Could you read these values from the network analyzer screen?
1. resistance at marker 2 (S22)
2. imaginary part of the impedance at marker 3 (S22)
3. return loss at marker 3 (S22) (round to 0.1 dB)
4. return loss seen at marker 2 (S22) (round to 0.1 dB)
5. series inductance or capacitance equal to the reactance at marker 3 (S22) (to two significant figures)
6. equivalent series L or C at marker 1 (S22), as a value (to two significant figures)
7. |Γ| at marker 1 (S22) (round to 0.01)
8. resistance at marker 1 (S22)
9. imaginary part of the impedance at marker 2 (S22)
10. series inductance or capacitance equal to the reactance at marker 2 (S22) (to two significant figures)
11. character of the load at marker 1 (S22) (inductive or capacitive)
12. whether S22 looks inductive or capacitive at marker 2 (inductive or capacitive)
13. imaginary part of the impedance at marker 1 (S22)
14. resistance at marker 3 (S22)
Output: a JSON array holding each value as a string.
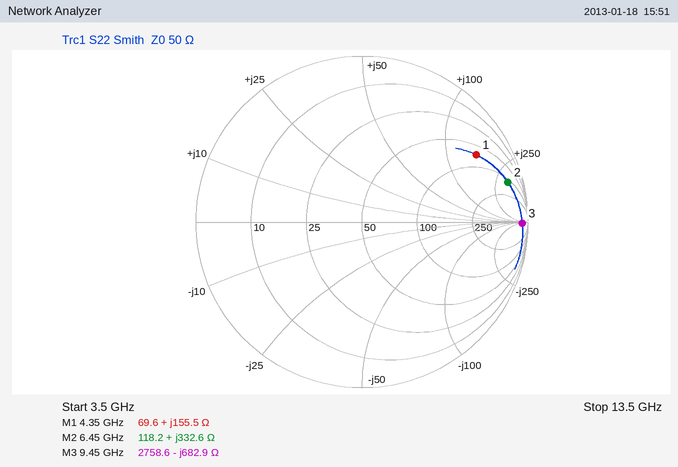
["118.2 Ω", "-682.9 Ω", "0.3 dB", "0.8 dB", "25 fF", "5.7 nH", "0.80", "69.6 Ω", "+332.6 Ω", "8.2 nH", "inductive", "inductive", "+155.5 Ω", "2758.6 Ω"]
